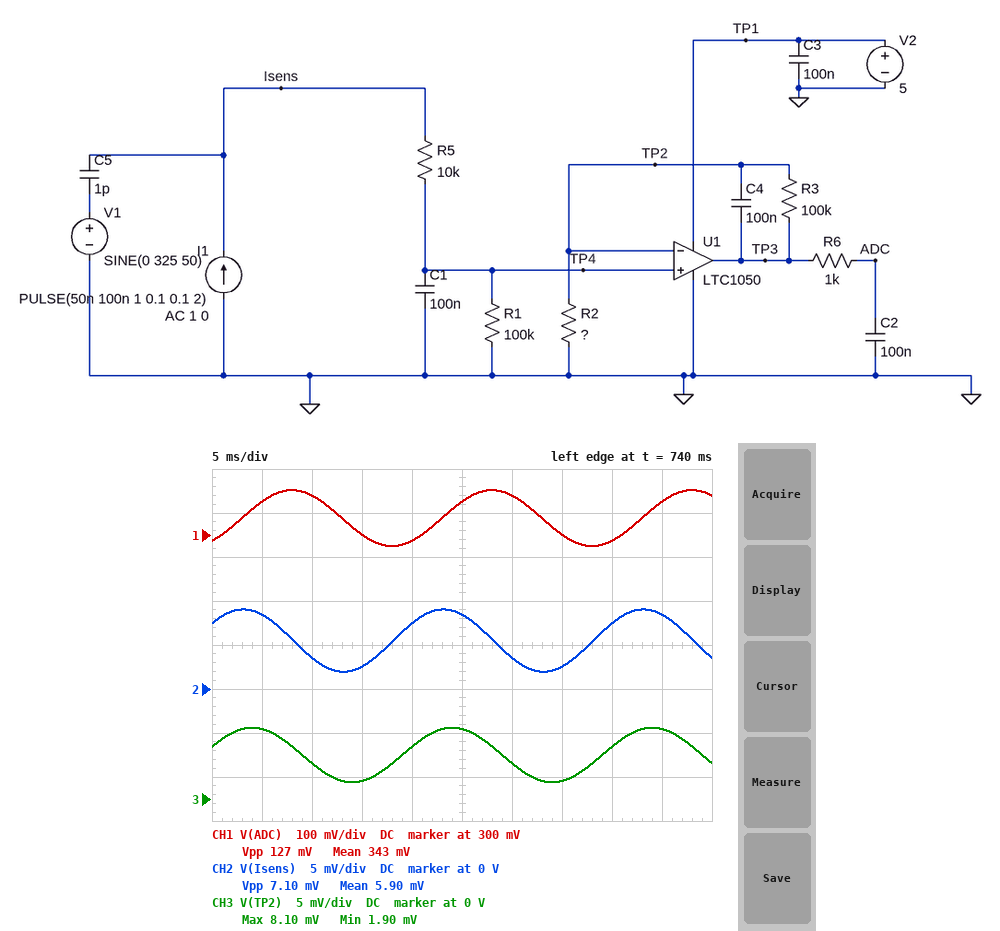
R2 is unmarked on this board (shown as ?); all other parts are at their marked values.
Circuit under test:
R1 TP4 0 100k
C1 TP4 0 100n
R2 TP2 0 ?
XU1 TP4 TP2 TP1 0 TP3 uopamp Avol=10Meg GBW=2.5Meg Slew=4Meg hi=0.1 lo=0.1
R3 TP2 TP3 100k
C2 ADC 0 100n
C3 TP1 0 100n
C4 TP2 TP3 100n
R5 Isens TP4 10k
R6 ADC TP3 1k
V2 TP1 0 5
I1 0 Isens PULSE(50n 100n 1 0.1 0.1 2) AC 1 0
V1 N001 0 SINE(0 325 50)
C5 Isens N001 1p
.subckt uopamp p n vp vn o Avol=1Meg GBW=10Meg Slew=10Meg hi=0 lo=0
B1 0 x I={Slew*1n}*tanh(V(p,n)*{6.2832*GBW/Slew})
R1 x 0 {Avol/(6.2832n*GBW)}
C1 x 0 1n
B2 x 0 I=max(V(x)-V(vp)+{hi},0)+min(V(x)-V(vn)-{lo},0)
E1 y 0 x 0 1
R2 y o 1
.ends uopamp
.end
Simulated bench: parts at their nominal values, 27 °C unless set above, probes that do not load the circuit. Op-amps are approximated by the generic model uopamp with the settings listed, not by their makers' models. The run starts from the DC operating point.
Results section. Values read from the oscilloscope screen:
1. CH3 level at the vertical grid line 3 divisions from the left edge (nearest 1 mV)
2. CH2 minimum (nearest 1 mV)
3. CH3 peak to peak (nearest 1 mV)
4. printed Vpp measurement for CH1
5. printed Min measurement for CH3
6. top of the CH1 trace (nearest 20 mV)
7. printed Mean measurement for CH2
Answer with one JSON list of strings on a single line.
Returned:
["2 mV", "2 mV", "6 mV", "127 mV", "1.90 mV", "400 mV", "5.90 mV"]
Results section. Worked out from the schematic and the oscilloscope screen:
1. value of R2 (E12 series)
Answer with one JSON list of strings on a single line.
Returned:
["1.5 kΩ"]
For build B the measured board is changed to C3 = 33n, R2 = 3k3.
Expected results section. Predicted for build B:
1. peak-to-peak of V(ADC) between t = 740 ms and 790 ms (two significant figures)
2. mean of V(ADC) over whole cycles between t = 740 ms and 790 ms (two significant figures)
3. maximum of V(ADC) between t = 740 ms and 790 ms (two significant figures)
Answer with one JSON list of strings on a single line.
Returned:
["59 mV", "160 mV", "190 mV"]
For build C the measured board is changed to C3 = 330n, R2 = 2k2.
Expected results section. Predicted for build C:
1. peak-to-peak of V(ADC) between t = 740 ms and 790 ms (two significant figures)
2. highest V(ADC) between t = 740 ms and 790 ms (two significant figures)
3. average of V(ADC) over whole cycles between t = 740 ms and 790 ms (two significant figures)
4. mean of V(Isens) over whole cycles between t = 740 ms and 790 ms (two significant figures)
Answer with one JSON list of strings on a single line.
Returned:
["87 mV", "280 mV", "230 mV", "5.5 mV"]
